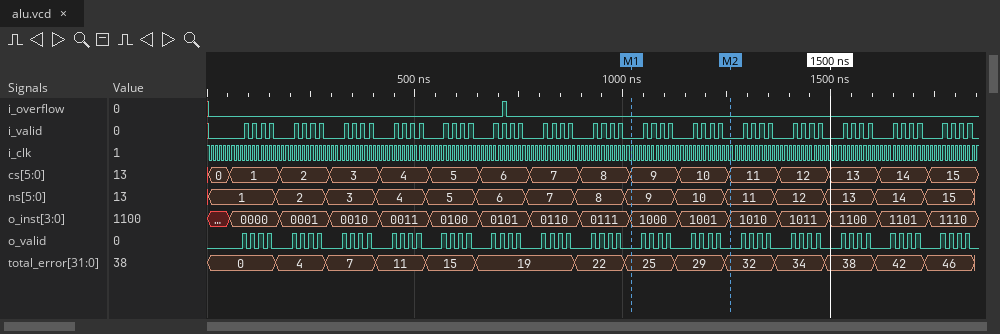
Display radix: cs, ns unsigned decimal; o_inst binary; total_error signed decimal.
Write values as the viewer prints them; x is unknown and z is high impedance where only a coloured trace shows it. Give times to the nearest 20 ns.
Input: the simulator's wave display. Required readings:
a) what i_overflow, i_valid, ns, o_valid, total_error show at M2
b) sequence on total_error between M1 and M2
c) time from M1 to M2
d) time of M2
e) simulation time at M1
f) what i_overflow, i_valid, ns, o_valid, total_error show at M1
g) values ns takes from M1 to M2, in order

i_overflow=0, i_valid=0, ns=11, o_valid=0, total_error=32
25, 29, 32
240 ns
1260 ns
1020 ns
i_overflow=0, i_valid=0, ns=9, o_valid=0, total_error=25
9, 10, 11
